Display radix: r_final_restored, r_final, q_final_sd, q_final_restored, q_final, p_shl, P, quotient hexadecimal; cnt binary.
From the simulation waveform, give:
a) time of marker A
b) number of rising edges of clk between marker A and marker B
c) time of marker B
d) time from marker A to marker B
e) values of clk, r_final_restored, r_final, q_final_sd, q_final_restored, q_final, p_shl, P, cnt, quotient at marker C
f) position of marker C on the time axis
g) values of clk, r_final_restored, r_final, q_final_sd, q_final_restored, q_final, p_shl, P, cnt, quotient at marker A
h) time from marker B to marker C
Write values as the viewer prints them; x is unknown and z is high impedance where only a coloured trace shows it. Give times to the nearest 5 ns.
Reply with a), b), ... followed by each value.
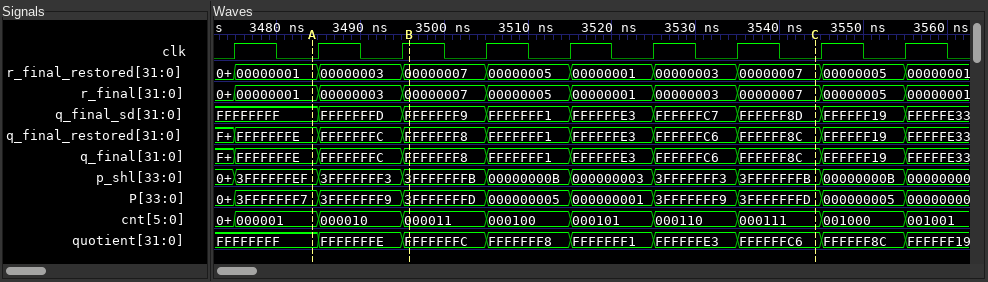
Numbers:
a) 3485 ns
b) 2
c) 3495 ns
d) 10 ns
e) clk=0, r_final_restored=00000007, r_final=00000007, q_final_sd=FFFFFF8D, q_final_restored=FFFFFF8C, q_final=FFFFFF8C, p_shl=3FFFFFFFB, P=3FFFFFFFD, cnt=000111, quotient=FFFFFFC6
f) 3545 ns
g) clk=0, r_final_restored=00000001, r_final=00000001, q_final_sd=FFFFFFFF, q_final_restored=FFFFFFFE, q_final=FFFFFFFE, p_shl=3FFFFFFEF, P=3FFFFFFF7, cnt=000001, quotient=FFFFFFFF
h) 50 ns
